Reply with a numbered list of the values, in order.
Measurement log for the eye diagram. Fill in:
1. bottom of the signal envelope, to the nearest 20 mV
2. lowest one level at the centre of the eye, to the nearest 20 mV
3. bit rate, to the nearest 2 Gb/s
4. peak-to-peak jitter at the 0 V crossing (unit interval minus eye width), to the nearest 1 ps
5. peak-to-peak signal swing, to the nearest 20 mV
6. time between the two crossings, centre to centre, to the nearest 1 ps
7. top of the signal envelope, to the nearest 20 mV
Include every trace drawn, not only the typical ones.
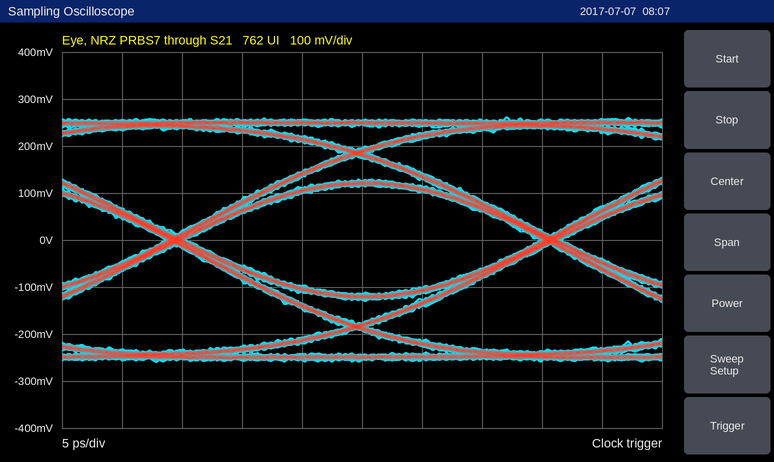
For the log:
1. -260 mV
2. 120 mV
3. 32 Gb/s
4. 2 ps
5. 520 mV
6. 31 ps
7. 260 mV
